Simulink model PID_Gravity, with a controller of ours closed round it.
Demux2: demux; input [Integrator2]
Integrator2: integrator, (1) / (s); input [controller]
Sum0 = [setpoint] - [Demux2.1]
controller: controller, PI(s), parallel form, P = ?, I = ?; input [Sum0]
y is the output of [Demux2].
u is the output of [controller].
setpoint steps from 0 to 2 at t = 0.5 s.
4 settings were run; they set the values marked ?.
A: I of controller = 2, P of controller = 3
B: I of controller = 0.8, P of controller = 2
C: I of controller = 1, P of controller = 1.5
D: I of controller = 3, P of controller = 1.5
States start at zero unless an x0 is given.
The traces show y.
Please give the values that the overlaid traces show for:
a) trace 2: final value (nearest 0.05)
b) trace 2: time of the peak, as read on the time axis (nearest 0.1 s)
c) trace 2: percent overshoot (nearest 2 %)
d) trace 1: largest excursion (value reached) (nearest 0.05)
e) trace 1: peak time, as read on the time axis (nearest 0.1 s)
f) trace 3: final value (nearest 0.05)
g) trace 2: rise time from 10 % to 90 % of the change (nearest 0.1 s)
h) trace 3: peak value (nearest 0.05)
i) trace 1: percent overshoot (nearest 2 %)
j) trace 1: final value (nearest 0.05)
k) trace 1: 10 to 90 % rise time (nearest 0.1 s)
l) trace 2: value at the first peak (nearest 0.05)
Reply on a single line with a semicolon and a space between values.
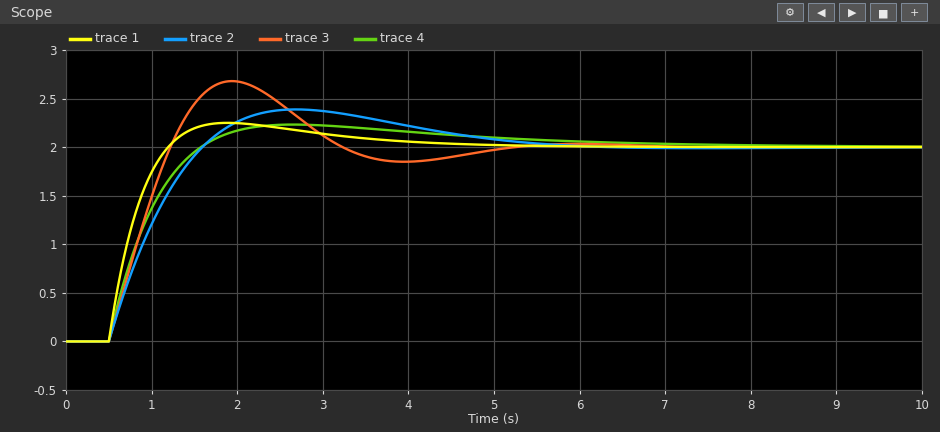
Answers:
2.00; 2.7 s; 20 %; 2.25; 1.9 s; 2.00; 0.8 s; 2.70; 12 %; 2.00; 0.5 s; 2.40
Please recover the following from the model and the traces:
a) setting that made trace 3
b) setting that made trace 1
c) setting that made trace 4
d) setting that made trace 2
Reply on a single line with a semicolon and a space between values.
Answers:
D; A; B; C
